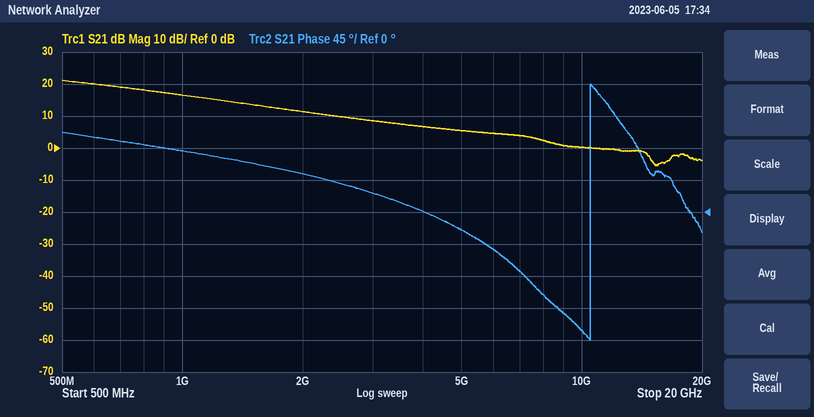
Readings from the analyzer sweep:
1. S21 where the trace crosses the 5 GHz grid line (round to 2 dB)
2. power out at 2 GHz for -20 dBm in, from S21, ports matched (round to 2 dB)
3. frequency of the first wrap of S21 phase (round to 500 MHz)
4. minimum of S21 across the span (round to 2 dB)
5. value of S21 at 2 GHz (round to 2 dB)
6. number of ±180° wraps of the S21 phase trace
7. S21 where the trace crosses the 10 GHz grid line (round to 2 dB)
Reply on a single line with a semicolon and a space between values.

6 dB; -8 dBm; 10.5 GHz; -6 dB; 12 dB; 1; 0 dB
